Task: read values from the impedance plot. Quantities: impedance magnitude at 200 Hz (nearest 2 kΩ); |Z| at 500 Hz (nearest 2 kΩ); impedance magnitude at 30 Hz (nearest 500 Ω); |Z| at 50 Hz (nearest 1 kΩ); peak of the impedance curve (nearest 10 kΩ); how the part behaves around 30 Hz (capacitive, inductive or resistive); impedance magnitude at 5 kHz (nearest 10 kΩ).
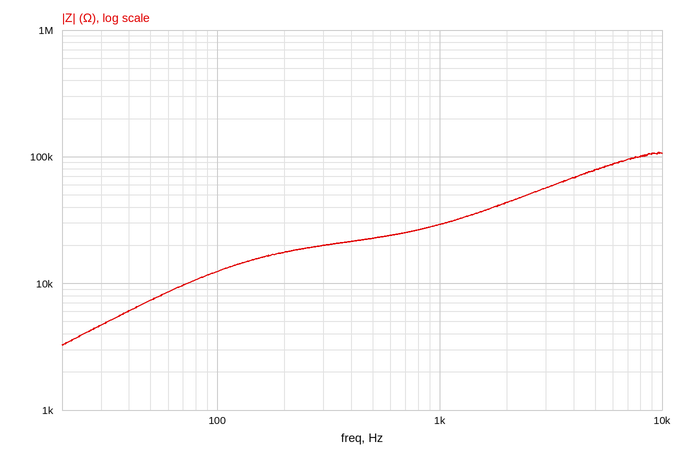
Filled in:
18 kΩ
22 kΩ
4.5 kΩ
7 kΩ
110 kΩ
inductive
80 kΩ
